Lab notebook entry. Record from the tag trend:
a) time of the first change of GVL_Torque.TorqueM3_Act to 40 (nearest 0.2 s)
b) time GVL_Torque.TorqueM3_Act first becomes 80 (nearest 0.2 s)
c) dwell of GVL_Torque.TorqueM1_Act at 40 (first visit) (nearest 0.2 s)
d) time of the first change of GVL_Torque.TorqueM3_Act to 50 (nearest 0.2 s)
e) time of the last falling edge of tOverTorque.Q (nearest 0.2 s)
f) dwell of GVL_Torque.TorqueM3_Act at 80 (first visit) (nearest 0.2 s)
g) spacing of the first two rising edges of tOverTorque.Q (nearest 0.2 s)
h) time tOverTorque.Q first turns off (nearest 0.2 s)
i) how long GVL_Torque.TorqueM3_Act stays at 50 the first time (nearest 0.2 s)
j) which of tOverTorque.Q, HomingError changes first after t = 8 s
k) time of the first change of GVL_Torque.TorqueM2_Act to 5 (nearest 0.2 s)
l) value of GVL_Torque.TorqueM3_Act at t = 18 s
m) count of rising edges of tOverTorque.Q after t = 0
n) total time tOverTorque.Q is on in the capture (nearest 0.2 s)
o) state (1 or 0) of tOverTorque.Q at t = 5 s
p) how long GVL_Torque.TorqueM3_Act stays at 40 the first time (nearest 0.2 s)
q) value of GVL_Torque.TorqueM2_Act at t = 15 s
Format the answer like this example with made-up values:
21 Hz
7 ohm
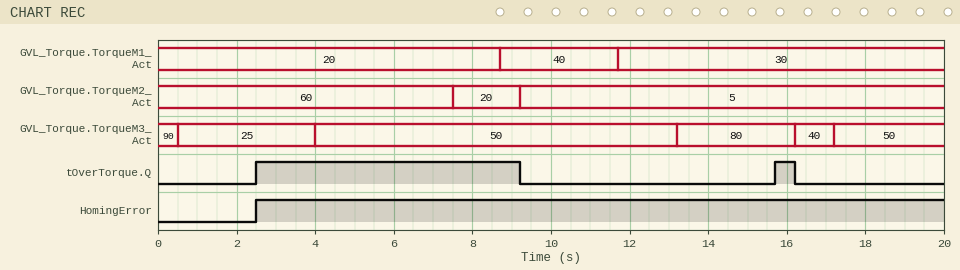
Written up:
16.2 s
13.2 s
3.0 s
4.0 s
16.2 s
3.0 s
13.2 s
9.2 s
9.2 s
tOverTorque.Q
9.2 s
50
2
7.2 s
1
1.0 s
5
